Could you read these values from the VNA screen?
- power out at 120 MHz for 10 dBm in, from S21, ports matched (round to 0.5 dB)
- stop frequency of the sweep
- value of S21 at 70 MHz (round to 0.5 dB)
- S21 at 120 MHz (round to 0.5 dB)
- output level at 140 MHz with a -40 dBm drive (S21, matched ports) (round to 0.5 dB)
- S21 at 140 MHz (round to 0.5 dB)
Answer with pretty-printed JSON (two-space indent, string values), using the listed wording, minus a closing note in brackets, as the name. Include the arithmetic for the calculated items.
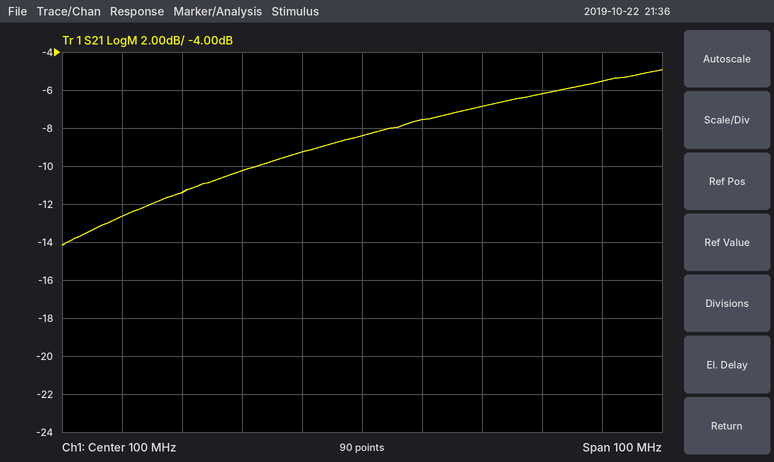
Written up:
{
  "power out at 120 MHz for 10 dBm in, from S21, ports matched": "10 dBm + (-7.0 dB) = 3.0 dBm",
  "stop frequency of the sweep": "150 MHz",
  "value of S21 at 70 MHz": "-11.5 dB",
  "S21 at 120 MHz": "-7.0 dB",
  "output level at 140 MHz with a -40 dBm drive (S21, matched ports)": "-40 dBm + (-5.5 dB) = -45.5 dBm",
  "S21 at 140 MHz": "-5.5 dB"
}
